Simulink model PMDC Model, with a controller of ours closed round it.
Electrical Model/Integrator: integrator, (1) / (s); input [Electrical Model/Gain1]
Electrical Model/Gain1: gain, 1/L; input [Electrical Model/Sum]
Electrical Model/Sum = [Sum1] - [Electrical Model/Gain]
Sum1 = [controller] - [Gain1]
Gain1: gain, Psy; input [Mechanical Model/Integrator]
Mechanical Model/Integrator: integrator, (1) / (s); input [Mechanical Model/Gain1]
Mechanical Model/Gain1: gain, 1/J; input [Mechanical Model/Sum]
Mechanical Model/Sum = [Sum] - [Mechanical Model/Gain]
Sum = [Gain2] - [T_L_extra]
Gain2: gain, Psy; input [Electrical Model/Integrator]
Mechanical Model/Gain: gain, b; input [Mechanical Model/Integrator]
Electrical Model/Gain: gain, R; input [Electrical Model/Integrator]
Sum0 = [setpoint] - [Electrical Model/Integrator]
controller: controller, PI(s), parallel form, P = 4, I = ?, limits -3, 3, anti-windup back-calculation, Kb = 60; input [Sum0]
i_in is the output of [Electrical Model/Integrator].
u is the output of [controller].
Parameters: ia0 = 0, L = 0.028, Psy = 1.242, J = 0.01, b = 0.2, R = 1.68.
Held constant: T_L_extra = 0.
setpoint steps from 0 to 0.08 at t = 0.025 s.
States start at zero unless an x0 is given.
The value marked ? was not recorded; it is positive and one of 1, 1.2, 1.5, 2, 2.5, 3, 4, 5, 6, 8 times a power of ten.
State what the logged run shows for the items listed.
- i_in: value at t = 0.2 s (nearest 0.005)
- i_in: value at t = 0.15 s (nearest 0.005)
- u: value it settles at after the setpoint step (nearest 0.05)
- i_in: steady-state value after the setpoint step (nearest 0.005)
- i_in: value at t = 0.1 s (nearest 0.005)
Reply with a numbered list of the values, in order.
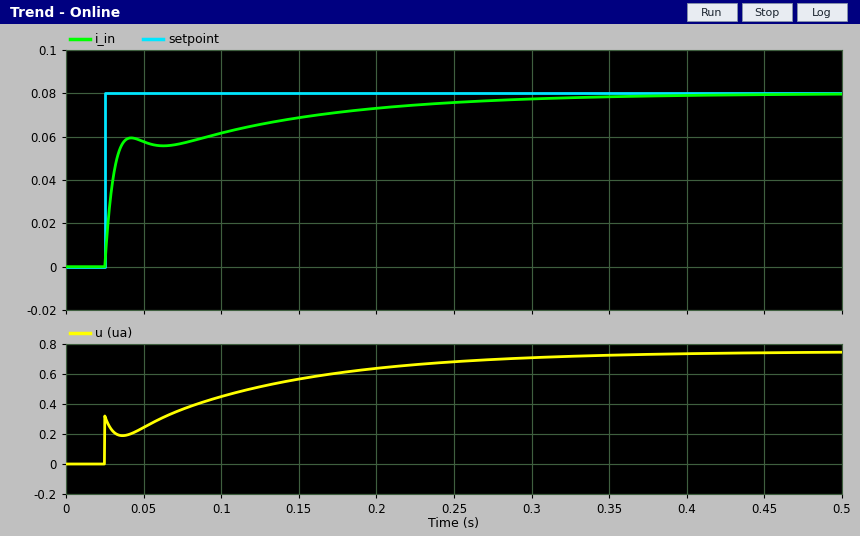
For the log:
1. 0.075
2. 0.070
3. 0.75
4. 0.080
5. 0.060
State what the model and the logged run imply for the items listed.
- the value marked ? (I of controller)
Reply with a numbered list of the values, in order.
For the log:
1. 200
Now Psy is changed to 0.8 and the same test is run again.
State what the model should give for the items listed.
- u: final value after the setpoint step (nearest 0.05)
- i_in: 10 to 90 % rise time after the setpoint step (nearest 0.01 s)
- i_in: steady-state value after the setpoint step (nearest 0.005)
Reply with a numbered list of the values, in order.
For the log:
1. 0.40
2. 0.09 s
3. 0.080
